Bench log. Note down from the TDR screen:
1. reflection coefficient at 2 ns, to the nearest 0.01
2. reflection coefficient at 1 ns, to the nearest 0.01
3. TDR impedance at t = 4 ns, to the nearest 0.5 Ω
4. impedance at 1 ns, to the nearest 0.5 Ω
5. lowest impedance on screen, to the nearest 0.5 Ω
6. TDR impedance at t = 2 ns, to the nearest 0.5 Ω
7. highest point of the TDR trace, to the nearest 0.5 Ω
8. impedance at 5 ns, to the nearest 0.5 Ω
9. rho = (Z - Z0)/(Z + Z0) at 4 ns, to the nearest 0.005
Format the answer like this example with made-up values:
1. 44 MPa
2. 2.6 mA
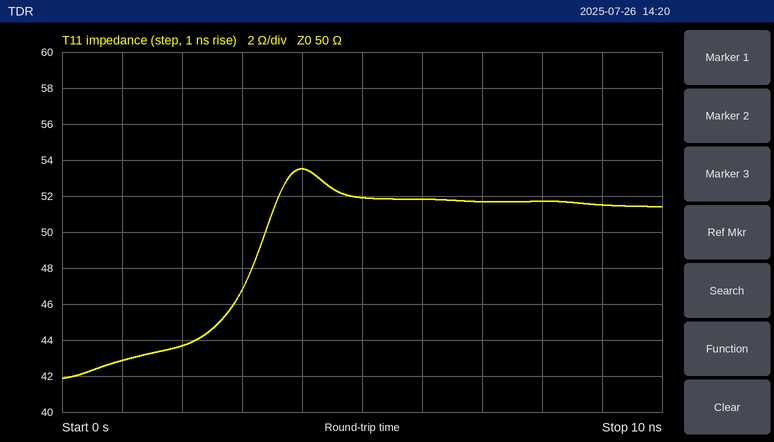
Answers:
1. -0.07
2. -0.08
3. 53.5 Ω
4. 43.0 Ω
5. 42.0 Ω
6. 43.5 Ω
7. 53.5 Ω
8. 52.0 Ω
9. +0.035
